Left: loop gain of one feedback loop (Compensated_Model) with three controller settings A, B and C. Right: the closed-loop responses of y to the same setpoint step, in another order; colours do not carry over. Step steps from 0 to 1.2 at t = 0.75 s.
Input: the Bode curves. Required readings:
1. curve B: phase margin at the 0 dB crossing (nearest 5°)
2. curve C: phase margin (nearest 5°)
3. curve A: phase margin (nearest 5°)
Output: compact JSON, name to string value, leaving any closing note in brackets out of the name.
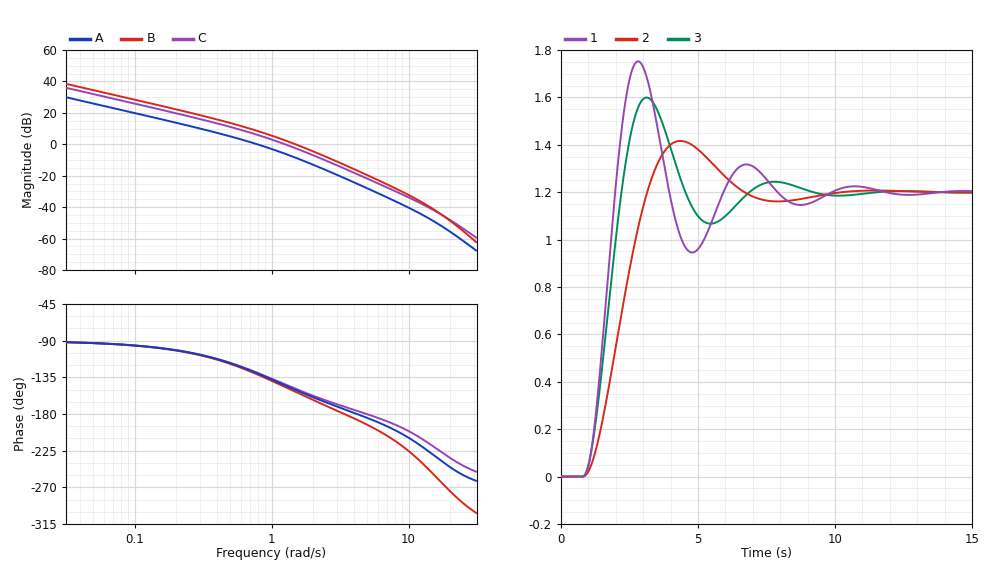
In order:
{"curve B: phase margin at the 0 dB crossing": "25°", "curve C: phase margin": "35°", "curve A: phase margin": "50°"}
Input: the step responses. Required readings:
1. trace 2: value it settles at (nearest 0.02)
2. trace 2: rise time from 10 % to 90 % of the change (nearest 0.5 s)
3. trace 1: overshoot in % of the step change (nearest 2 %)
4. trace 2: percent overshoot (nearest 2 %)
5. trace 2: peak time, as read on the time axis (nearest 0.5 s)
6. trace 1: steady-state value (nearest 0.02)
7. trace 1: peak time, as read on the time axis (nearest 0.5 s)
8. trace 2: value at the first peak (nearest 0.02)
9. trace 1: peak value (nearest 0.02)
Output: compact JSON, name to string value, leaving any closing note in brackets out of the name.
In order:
{"trace 2: value it settles at": "1.20", "trace 2: rise time from 10 % to 90 % of the change": "1.5 s", "trace 1: overshoot in % of the step change": "46 %", "trace 2: percent overshoot": "18 %", "trace 2: peak time, as read on the time axis": "4.5 s", "trace 1: steady-state value": "1.20", "trace 1: peak time, as read on the time axis": "3.0 s", "trace 2: value at the first peak": "1.42", "trace 1: peak value": "1.76"}
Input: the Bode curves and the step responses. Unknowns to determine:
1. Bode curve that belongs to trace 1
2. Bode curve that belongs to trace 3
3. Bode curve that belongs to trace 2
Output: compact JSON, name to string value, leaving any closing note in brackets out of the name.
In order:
{"Bode curve that belongs to trace 1": "B", "Bode curve that belongs to trace 3": "C", "Bode curve that belongs to trace 2": "A"}
